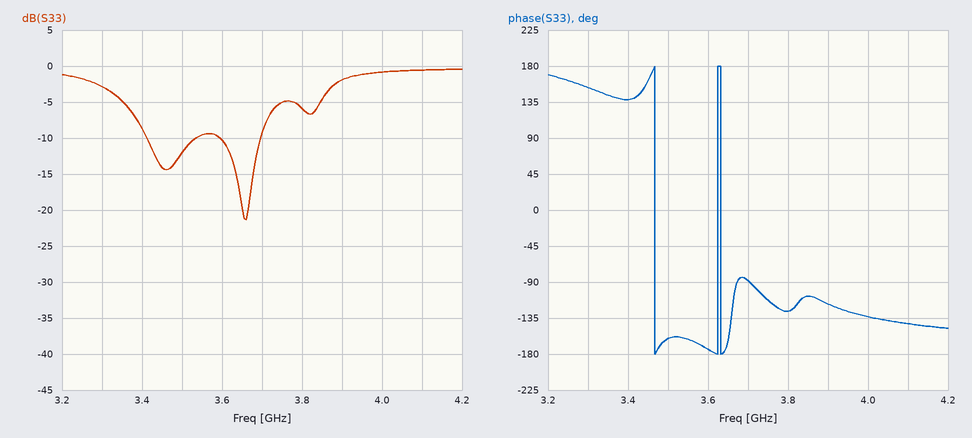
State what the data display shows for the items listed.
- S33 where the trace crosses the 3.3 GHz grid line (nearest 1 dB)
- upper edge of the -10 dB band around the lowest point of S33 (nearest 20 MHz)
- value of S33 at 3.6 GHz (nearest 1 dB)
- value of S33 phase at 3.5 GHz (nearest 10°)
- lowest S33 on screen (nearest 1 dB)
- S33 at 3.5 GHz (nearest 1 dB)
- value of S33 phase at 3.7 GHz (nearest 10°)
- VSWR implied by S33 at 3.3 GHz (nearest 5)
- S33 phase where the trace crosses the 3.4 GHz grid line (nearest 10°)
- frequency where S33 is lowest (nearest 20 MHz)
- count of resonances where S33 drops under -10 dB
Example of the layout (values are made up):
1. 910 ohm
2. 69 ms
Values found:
1. -3 dB
2. 3.70 GHz
3. -10 dB
4. -160°
5. -21 dB
6. -12 dB
7. -90°
8. 5
9. 140°
10. 3.66 GHz
11. 2
